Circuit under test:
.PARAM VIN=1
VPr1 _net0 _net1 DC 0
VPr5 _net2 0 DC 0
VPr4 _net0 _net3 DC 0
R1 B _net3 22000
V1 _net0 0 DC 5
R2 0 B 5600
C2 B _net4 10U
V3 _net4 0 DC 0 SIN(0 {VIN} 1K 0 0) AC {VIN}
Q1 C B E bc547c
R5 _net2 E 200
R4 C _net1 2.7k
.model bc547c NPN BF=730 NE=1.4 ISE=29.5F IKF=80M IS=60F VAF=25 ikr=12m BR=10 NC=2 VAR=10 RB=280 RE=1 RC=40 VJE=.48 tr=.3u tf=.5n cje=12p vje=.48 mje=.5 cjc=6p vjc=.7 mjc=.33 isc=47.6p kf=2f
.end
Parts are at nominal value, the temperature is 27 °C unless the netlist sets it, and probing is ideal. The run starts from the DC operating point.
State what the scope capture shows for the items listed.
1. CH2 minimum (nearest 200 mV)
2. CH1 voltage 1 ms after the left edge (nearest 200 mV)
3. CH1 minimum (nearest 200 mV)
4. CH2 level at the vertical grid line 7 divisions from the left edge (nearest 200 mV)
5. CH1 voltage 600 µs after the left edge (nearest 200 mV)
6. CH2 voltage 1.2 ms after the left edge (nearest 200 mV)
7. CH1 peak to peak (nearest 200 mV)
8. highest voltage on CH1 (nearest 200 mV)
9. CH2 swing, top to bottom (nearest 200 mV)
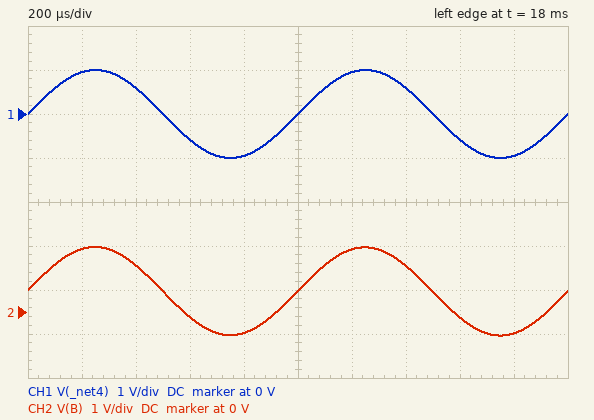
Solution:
-600 mV
0 V
-1.0 V
1.0 V
-600 mV
1.4 V
2.0 V
1.0 V
2.0 V
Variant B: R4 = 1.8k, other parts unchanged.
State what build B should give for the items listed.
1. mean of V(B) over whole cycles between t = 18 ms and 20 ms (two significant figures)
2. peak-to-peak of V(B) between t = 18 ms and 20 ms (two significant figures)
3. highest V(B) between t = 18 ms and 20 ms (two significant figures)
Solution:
580 mV
2.0 V
1.6 V
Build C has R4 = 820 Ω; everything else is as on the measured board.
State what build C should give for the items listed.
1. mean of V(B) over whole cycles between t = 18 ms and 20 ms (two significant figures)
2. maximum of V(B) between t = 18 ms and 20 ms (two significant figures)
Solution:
840 mV
1.8 V
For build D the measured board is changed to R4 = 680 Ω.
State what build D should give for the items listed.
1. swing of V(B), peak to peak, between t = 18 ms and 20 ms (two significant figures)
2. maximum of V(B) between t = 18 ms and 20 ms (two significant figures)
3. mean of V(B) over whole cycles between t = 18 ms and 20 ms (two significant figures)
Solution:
2.0 V
1.9 V
910 mV
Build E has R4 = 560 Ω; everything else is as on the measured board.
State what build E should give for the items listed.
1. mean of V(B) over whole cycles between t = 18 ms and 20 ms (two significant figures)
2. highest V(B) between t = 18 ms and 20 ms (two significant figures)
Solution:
970 mV
2.0 V
